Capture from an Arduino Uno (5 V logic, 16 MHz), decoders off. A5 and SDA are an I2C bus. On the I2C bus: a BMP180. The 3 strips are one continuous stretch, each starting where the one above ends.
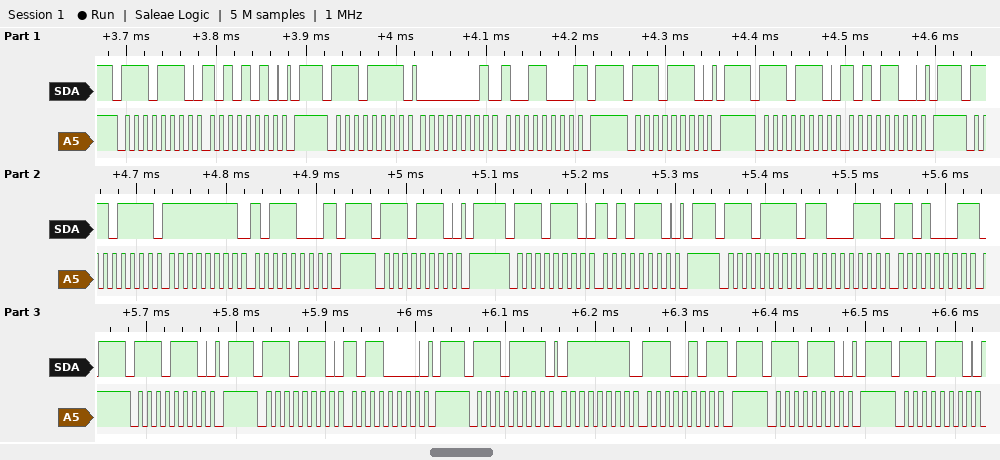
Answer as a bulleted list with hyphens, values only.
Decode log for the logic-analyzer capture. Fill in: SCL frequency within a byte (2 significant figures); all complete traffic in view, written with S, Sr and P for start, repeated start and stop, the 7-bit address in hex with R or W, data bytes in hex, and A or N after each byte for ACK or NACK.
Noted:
- 100 kHz
- S 77W A AA A P S 77R A 01 A 98 N P S 77W A P S 77W A AC A P S 77R A FF A B8 N P S 77W A P S 77W A AE A P S 77R A C7 A D1 N P S 77W A P S 77W A B0 A P S 77R A 7F A E5 N P S 77W A P S 77W A
